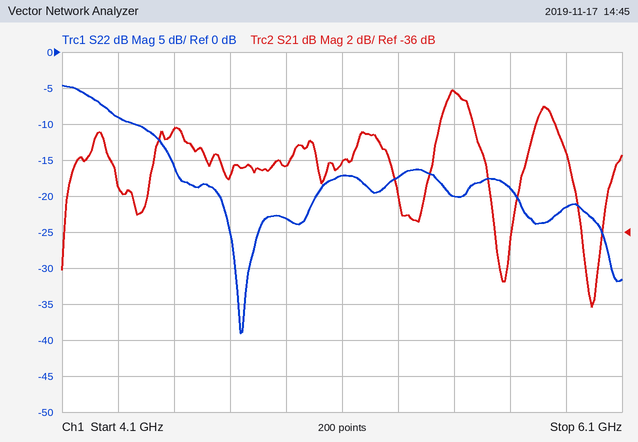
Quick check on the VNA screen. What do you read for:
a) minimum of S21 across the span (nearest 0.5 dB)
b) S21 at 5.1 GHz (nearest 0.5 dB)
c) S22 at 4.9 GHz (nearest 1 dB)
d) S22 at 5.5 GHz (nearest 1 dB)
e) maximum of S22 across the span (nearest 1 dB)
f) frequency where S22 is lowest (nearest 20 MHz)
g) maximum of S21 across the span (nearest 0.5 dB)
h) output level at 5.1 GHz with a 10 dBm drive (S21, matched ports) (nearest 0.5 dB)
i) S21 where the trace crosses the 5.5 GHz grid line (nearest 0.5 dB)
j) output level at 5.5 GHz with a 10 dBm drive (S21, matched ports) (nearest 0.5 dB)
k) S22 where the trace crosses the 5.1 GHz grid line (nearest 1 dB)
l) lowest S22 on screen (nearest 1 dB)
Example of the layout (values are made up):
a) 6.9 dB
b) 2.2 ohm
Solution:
a) -40.0 dB
b) -32.0 dB
c) -23 dB
d) -20 dB
e) -5 dB
f) 4.74 GHz
g) -28.0 dB
h) -22.0 dBm
i) -28.0 dB
j) -18.0 dBm
k) -17 dB
l) -39 dB
